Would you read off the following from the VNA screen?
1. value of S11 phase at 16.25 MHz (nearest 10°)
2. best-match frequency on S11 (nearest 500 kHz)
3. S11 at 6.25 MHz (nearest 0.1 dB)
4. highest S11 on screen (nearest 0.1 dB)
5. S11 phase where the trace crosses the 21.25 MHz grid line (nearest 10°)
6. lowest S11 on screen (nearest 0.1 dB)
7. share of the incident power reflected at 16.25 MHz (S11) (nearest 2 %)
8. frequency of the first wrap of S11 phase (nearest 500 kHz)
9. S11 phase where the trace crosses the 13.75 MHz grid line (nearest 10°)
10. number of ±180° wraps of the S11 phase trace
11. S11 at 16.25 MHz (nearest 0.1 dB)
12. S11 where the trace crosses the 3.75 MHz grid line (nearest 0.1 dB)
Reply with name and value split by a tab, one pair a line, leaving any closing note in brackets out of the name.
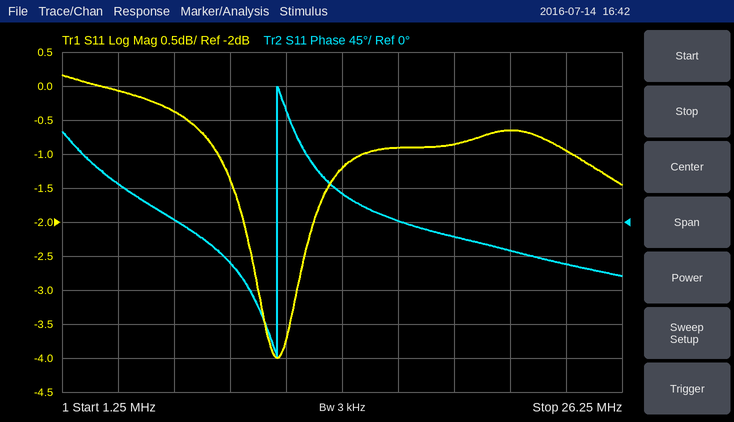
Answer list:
value of S11 phase at 16.25 MHz	0°
best-match frequency on S11	11.0 MHz
S11 at 6.25 MHz	-0.4 dB
highest S11 on screen	0.2 dB
S11 phase where the trace crosses the 21.25 MHz grid line	-40°
lowest S11 on screen	-4.0 dB
share of the incident power reflected at 16.25 MHz (S11)	82 %
frequency of the first wrap of S11 phase	11.0 MHz
S11 phase where the trace crosses the 13.75 MHz grid line	40°
number of ±180° wraps of the S11 phase trace	1
S11 at 16.25 MHz	-0.9 dB
S11 where the trace crosses the 3.75 MHz grid line	-0.1 dB
